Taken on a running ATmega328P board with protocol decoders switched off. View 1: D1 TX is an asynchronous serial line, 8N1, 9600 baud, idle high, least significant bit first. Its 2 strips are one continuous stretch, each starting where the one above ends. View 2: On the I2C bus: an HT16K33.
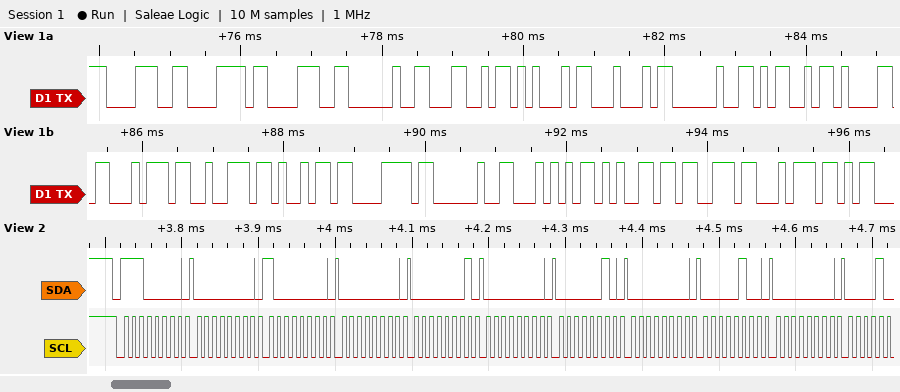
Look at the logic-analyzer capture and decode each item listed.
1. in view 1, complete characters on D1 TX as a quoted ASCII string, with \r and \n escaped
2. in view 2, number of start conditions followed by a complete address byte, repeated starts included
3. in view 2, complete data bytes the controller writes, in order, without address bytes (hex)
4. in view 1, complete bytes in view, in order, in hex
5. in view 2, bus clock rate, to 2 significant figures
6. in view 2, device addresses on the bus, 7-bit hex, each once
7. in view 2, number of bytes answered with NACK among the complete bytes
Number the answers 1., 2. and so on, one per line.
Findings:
1. "8x8 LED Matrix Test"
2. 1
3. 00 80 00 01 00 02 00 04 00
4. 38 78 38 20 4C 45 44 20 4D 61 74 72 69 78 20 54 65 73 74
5. 100 kHz
6. 0x70
7. 0
